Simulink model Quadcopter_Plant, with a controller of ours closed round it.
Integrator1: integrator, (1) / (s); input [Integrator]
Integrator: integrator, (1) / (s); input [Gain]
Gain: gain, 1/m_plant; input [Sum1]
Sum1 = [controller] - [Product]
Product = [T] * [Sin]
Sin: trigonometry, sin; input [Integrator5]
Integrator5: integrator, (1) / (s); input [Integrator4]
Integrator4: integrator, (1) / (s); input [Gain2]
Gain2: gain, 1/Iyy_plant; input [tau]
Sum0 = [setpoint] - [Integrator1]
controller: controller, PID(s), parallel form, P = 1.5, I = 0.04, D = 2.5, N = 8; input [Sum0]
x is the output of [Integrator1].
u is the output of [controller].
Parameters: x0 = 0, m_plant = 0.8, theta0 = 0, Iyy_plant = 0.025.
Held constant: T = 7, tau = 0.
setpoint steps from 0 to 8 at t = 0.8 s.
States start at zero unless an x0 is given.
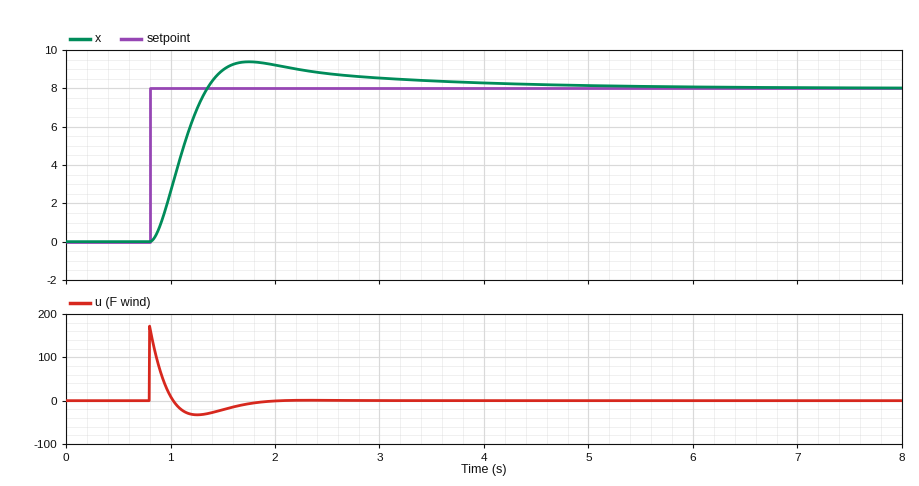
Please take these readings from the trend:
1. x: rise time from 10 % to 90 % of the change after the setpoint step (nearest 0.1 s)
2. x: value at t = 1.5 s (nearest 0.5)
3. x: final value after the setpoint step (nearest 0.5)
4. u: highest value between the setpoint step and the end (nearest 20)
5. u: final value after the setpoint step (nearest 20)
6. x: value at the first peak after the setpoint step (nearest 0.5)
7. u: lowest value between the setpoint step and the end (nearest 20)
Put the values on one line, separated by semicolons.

0.4 s; 9.0; 8.0; 180; 0; 9.5; -40
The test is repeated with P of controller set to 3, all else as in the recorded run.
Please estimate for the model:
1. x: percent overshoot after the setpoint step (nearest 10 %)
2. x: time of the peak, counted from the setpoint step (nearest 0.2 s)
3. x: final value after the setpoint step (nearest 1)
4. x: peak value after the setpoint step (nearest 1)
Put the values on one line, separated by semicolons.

30 %; 0.8 s; 8; 10
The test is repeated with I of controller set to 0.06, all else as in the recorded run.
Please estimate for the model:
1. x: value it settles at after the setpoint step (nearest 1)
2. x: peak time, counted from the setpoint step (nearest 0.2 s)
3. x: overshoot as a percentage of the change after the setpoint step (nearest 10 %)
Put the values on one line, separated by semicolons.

8; 1.0 s; 20 %
